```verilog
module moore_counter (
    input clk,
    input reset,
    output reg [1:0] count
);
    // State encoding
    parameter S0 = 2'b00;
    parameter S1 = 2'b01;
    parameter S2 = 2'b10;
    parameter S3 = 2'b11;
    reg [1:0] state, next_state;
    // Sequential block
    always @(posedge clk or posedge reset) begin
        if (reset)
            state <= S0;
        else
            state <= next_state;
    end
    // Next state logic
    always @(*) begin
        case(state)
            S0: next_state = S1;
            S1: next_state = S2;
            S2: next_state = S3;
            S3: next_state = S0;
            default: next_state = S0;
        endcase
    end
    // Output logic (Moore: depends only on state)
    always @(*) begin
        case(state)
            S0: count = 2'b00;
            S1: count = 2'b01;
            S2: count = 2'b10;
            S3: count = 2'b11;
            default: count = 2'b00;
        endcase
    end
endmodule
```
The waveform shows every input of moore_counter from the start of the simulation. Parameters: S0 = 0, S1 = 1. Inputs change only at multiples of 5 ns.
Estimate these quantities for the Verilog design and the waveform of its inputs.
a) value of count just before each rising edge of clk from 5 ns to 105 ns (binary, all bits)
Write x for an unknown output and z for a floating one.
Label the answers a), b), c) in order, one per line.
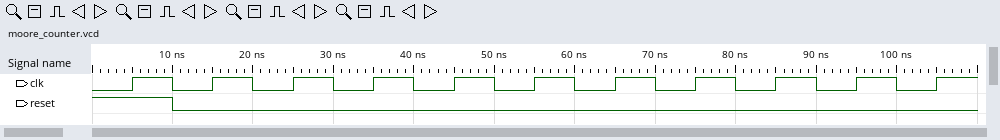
a) 00, 00, 01, 10, 11, 00, 01, 10, 11, 00, 01
